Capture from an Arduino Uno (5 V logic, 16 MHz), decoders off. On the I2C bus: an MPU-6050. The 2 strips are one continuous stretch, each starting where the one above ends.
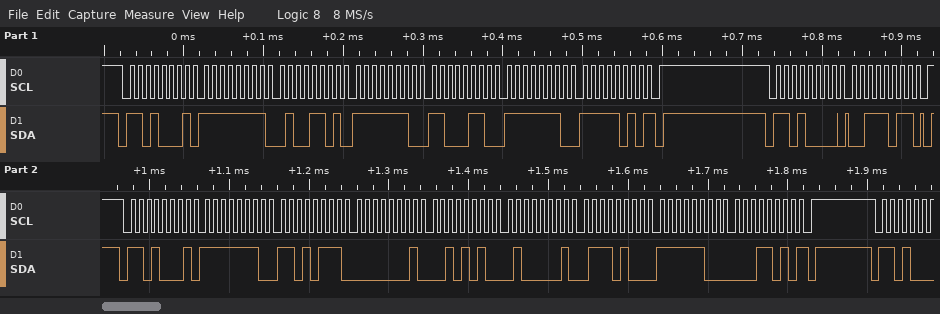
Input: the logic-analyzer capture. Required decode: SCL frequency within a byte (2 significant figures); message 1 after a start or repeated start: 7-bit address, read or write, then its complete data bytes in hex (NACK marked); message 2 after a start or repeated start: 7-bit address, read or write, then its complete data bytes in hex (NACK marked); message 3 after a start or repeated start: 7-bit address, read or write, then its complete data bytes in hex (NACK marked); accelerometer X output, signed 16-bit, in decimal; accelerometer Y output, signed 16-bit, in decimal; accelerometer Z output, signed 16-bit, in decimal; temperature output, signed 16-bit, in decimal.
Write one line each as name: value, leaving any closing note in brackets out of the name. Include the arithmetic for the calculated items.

SCL frequency within a byte: 100 kHz
message 1 after a start or repeated start: 7-bit address, read or write, then its complete data bytes in hex: 0x68 read: FF 4D FE C6 FE FA NACK
message 2 after a start or repeated start: 7-bit address, read or write, then its complete data bytes in hex: 0x68 write: 3B
message 3 after a start or repeated start: 7-bit address, read or write, then its complete data bytes in hex: 0x68 read: FE D7 01 2A 41 74 FC 1A NACK
accelerometer X output, signed 16-bit, in decimal: 0xFED7 = -297
accelerometer Y output, signed 16-bit, in decimal: 0x012A = 298
accelerometer Z output, signed 16-bit, in decimal: 0x4174 = 16756
temperature output, signed 16-bit, in decimal: 0xFC1A = -998
